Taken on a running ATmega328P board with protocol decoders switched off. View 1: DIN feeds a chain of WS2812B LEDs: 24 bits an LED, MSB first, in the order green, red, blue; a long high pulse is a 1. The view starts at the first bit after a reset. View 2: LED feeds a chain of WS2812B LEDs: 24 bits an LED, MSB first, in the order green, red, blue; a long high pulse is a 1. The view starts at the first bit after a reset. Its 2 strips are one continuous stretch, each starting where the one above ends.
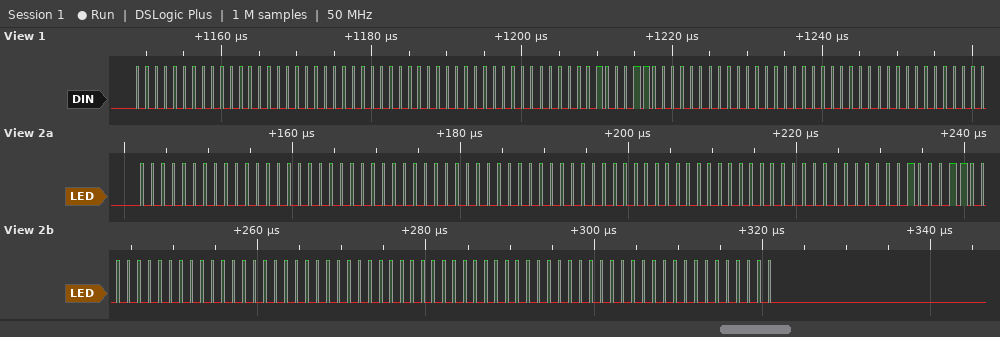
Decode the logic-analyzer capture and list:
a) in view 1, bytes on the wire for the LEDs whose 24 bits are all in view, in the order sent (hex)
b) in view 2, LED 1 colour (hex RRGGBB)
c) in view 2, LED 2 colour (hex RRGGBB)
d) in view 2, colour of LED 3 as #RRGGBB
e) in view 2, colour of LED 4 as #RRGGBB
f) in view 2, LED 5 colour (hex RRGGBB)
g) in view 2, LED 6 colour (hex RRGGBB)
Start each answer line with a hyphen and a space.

- 00 00 00 00 00 00 46 00 00
- #000000
- #000000
- #000000
- #004600
- #000000
- #000000
